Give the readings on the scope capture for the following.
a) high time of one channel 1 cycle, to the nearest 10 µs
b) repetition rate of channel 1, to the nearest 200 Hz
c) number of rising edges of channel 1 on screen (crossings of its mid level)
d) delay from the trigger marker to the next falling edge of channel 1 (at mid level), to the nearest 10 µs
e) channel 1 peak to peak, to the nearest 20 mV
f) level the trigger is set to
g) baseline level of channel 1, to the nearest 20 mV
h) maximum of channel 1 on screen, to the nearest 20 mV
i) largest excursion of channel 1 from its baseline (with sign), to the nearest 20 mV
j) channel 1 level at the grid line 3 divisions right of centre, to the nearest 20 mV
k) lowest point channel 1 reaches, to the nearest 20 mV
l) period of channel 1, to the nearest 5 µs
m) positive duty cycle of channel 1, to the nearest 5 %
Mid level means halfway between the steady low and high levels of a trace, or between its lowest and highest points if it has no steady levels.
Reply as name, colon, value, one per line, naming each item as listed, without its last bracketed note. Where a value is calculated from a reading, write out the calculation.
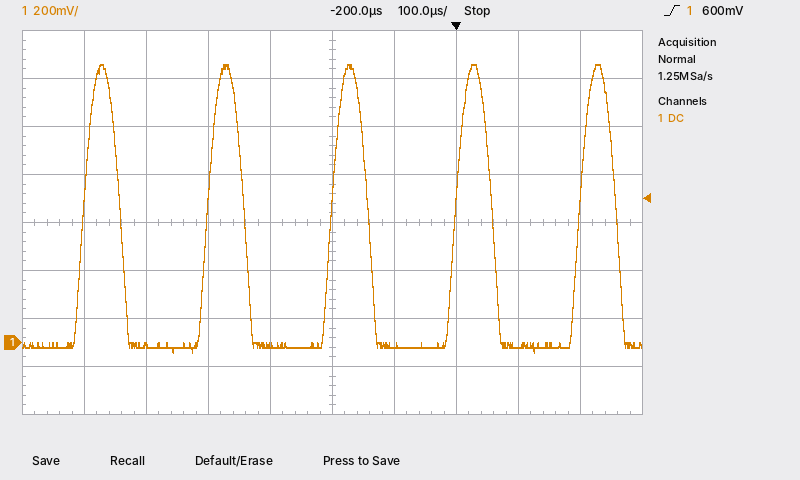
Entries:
high time of one channel 1 cycle, to the nearest 10 µs: 60 µs
repetition rate of channel 1, to the nearest 200 Hz: 1 / 200 µs ≈ 5.0 kHz
number of rising edges of channel 1 on screen: 5
delay from the trigger marker to the next falling edge of channel 1 (at mid level), to the nearest 10 µs: 60 µs
channel 1 peak to peak, to the nearest 20 mV: 1.16 V − (-40 mV) = 1.20 V
level the trigger is set to: 600 mV
baseline level of channel 1, to the nearest 20 mV: -20 mV
maximum of channel 1 on screen, to the nearest 20 mV: 1.16 V
largest excursion of channel 1 from its baseline (with sign), to the nearest 20 mV: 1.16 V − (-20 mV) = +1.18 V
channel 1 level at the grid line 3 divisions right of centre, to the nearest 20 mV: -20 mV
lowest point channel 1 reaches, to the nearest 20 mV: -40 mV
period of channel 1, to the nearest 5 µs: 200 µs
positive duty cycle of channel 1, to the nearest 5 %: 60 µs / 200 µs ≈ 30 %
